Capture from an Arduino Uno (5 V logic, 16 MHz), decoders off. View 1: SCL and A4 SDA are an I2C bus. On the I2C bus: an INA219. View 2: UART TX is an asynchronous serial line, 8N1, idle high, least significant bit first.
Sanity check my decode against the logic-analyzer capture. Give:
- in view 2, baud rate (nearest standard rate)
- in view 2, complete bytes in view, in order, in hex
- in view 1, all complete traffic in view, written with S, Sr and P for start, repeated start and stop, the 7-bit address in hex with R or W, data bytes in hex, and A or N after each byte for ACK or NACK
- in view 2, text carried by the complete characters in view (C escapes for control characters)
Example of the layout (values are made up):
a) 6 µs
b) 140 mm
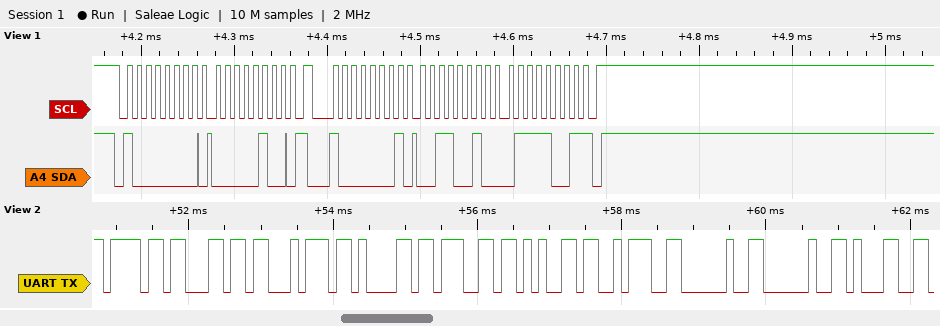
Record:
a) 9600 baud
b) 0x6F 0x6C 0x74 0x61 0x67 0x65 0x3A 0x20 0x20 0x31
c) S 40W A 04 A Sr 40R A 32 A 79 N P
d) "oltage:  1"
